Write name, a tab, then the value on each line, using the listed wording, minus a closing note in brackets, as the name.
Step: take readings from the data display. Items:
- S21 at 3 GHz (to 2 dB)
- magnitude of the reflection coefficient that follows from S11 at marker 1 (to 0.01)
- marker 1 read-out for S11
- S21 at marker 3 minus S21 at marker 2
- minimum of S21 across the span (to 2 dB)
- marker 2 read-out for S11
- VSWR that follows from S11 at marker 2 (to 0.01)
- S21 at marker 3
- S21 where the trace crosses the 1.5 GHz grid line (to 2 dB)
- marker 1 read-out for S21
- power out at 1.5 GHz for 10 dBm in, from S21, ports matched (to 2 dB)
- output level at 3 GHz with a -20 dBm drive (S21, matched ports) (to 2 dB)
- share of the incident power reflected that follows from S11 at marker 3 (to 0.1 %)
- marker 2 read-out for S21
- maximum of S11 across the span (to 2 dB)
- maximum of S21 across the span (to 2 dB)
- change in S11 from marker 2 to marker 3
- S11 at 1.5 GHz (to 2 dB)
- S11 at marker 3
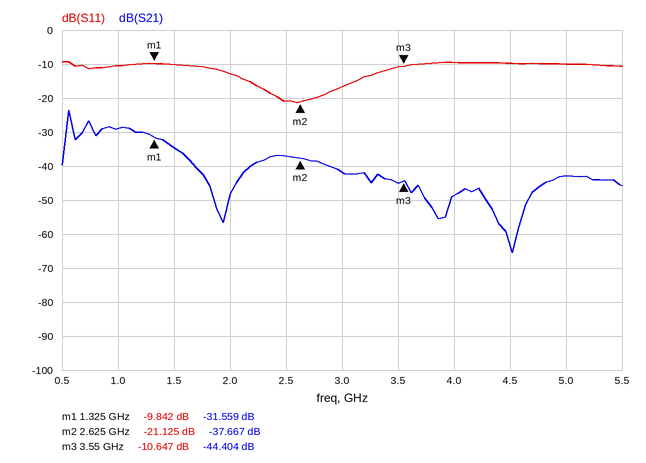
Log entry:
S21 at 3 GHz	-42 dB
magnitude of the reflection coefficient that follows from S11 at marker 1	0.32
marker 1 read-out for S11	-9.842 dB
S21 at marker 3 minus S21 at marker 2	-6.737 dB
minimum of S21 across the span	-66 dB
marker 2 read-out for S11	-21.125 dB
VSWR that follows from S11 at marker 2	1.19
S21 at marker 3	-44.404 dB
S21 where the trace crosses the 1.5 GHz grid line	-34 dB
marker 1 read-out for S21	-31.559 dB
power out at 1.5 GHz for 10 dBm in, from S21, ports matched	-24 dBm
output level at 3 GHz with a -20 dBm drive (S21, matched ports)	-62 dBm
share of the incident power reflected that follows from S11 at marker 3	8.6 %
marker 2 read-out for S21	-37.667 dB
maximum of S11 across the span	-10 dB
maximum of S21 across the span	-24 dB
change in S11 from marker 2 to marker 3	10.478 dB
S11 at 1.5 GHz	-10 dB
S11 at marker 3	-10.647 dB
